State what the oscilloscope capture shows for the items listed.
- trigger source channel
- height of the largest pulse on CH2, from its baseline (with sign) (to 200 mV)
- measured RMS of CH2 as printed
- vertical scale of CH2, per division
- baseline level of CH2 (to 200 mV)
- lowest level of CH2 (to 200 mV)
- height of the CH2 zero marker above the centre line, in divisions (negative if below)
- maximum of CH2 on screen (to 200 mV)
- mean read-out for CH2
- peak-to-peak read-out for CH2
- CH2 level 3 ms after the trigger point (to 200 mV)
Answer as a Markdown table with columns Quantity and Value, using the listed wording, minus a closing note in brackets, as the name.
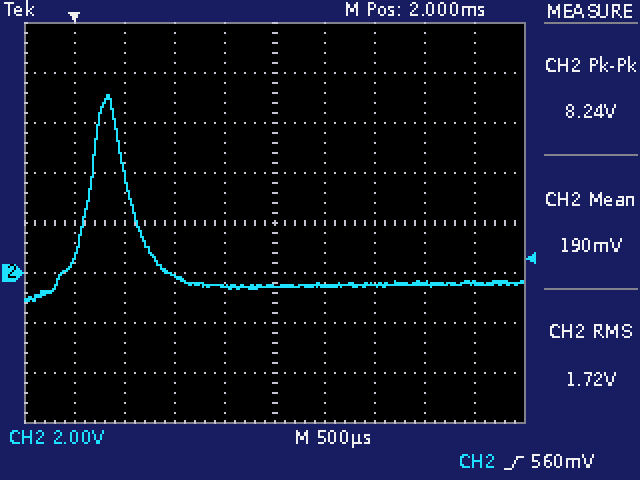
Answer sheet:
| Quantity | Value |
|---|---|
| trigger source channel | CH2 |
| height of the largest pulse on CH2, from its baseline (with sign) | +7.6 V |
| measured RMS of CH2 as printed | 1.72 V |
| vertical scale of CH2, per division | 2 V |
| baseline level of CH2 | -400 mV |
| lowest level of CH2 | -1.2 V |
| height of the CH2 zero marker above the centre line, in divisions | -1.0 div |
| maximum of CH2 on screen | 7.2 V |
| mean read-out for CH2 | 190 mV |
| peak-to-peak read-out for CH2 | 8.24 V |
| CH2 level 3 ms after the trigger point | -400 mV |
